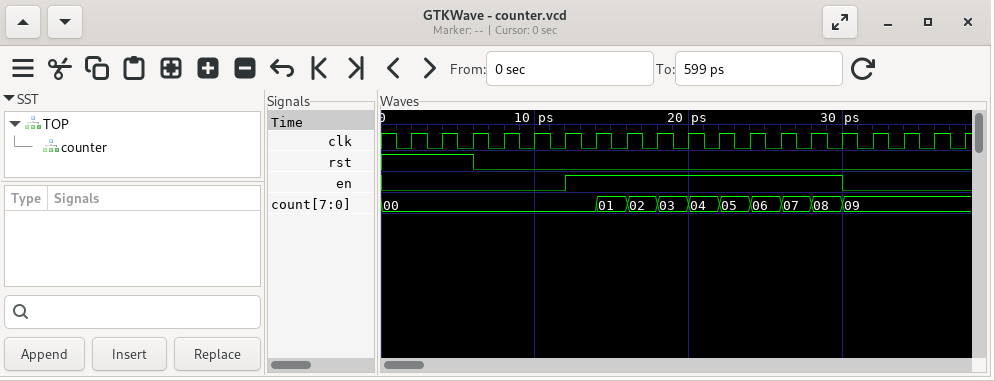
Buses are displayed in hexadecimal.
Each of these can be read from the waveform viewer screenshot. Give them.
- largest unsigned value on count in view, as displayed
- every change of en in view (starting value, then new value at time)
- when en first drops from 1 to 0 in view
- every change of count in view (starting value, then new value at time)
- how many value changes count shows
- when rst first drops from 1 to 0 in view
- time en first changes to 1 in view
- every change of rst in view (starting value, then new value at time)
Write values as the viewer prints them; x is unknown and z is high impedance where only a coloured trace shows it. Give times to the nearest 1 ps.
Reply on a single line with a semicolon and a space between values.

09; 0, 1 at 12 ps, 0 at 30 ps; 30 ps; 00, 01 at 14 ps, 02 at 16 ps, 03 at 18 ps, 04 at 20 ps, 05 at 22 ps, 06 at 24 ps, 07 at 26 ps, 08 at 28 ps, 09 at 30 ps; 9; 6 ps; 12 ps; 1, 0 at 6 ps
